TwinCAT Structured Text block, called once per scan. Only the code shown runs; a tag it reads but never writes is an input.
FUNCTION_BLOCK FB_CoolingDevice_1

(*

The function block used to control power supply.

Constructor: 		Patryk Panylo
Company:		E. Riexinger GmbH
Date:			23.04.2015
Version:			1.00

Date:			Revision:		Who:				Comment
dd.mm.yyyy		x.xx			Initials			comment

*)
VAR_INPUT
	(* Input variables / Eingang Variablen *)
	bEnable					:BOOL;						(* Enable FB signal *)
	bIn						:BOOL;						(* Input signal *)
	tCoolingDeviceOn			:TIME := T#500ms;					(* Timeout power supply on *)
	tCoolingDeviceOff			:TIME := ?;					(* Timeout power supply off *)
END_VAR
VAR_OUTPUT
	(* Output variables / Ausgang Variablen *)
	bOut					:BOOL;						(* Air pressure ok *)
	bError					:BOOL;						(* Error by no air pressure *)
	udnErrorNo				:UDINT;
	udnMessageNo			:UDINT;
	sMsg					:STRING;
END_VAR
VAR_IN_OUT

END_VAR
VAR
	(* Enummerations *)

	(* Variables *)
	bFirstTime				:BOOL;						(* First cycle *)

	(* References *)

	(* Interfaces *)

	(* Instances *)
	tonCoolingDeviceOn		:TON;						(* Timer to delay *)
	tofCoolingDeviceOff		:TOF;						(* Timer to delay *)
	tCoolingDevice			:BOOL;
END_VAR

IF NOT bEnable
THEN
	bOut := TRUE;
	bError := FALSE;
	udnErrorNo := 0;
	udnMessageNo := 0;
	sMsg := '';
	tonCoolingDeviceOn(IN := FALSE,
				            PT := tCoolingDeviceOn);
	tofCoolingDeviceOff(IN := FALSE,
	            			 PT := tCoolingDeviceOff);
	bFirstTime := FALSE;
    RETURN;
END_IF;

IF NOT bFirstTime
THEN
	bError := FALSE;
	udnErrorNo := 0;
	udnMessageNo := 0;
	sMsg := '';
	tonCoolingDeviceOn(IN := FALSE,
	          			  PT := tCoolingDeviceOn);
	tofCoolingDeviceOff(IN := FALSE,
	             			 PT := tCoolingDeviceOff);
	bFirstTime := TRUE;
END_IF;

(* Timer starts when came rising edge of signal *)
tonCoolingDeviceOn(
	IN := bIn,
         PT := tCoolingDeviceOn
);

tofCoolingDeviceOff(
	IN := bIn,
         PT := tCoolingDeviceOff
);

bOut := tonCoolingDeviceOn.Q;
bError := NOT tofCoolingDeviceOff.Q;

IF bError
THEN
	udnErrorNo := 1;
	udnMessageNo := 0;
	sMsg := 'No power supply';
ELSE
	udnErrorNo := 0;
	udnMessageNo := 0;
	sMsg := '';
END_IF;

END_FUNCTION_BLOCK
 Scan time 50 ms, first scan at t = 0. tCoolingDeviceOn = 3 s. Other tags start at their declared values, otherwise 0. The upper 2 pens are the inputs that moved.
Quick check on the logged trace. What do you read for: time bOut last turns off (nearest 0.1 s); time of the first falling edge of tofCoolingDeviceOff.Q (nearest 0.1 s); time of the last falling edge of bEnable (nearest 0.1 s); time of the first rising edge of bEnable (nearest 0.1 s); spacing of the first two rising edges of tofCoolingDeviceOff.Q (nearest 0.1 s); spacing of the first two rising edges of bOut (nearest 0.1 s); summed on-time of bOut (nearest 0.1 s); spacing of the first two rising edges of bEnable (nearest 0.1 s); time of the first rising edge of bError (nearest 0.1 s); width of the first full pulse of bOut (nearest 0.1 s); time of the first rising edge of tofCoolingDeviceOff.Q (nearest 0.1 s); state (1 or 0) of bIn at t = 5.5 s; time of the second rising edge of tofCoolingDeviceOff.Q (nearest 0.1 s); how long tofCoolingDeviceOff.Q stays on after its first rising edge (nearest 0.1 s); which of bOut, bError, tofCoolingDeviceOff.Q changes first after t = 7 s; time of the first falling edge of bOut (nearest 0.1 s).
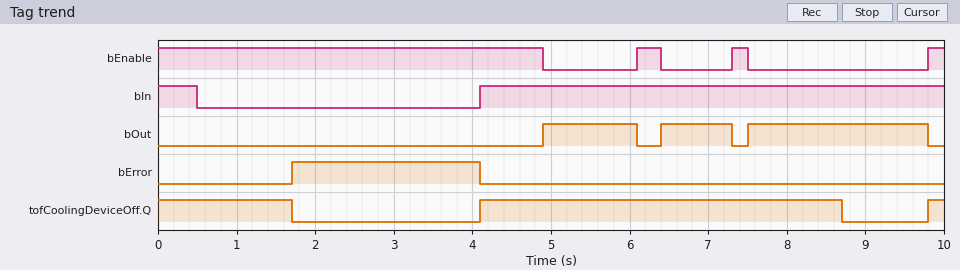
9.8 s
1.7 s
7.5 s
6.1 s
5.7 s
1.5 s
4.4 s
1.2 s
1.7 s
1.2 s
4.1 s
1
9.8 s
4.6 s
bOut
6.1 s
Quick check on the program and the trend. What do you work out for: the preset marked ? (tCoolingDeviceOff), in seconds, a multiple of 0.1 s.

1.2 s
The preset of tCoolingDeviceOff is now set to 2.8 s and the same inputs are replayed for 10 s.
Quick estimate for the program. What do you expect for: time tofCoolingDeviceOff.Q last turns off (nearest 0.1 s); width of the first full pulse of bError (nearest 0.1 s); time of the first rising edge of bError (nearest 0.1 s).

3.3 s
0.8 s
3.3 s
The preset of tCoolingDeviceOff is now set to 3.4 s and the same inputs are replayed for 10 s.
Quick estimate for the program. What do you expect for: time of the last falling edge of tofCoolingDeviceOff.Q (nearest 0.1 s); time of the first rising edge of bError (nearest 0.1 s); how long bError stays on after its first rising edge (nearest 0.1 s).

3.9 s
3.9 s
0.2 s
